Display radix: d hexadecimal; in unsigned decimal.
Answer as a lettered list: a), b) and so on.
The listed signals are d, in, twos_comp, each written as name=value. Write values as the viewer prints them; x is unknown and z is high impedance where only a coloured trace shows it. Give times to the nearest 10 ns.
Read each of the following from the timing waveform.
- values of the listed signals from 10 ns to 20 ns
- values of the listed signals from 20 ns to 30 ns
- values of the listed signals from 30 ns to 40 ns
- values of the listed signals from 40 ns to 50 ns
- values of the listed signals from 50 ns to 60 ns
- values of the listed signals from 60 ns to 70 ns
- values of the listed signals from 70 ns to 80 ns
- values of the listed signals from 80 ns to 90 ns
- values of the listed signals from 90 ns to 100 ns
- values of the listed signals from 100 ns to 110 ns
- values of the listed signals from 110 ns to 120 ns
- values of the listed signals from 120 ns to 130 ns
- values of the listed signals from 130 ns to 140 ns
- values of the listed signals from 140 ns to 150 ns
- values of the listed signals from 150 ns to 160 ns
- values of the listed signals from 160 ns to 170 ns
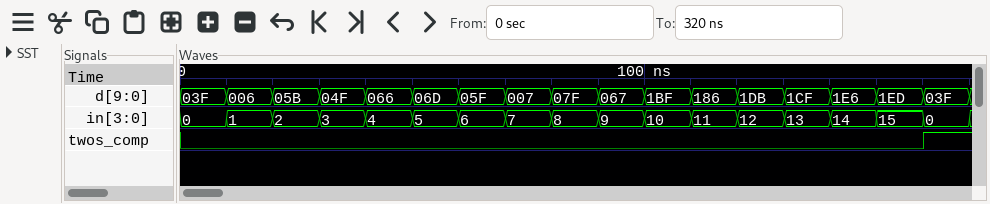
a) d=006, in=1, twos_comp=0
b) d=05B, in=2, twos_comp=0
c) d=04F, in=3, twos_comp=0
d) d=066, in=4, twos_comp=0
e) d=06D, in=5, twos_comp=0
f) d=05F, in=6, twos_comp=0
g) d=007, in=7, twos_comp=0
h) d=07F, in=8, twos_comp=0
i) d=067, in=9, twos_comp=0
j) d=1BF, in=10, twos_comp=0
k) d=186, in=11, twos_comp=0
l) d=1DB, in=12, twos_comp=0
m) d=1CF, in=13, twos_comp=0
n) d=1E6, in=14, twos_comp=0
o) d=1ED, in=15, twos_comp=0
p) d=03F, in=0, twos_comp=1
